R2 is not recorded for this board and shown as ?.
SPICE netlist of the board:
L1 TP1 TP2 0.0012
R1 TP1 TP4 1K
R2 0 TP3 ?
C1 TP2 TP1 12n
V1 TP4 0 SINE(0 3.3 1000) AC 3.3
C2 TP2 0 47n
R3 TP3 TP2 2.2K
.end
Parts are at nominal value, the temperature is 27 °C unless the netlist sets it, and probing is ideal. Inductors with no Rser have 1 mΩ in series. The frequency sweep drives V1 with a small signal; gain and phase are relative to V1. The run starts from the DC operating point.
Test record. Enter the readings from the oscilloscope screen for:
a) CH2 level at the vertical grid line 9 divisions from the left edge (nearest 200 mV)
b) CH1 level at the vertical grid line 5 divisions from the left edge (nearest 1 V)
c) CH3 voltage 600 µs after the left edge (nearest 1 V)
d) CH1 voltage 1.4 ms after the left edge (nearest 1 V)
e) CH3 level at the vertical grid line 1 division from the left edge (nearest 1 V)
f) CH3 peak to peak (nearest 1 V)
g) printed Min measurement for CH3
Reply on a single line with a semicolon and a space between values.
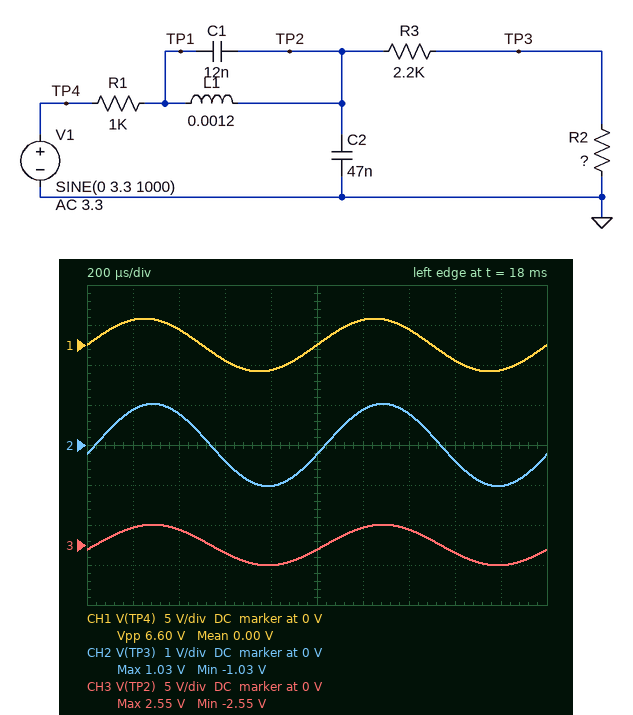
-1.0 V; 0 V; -1 V; 2 V; 2 V; 5 V; -2.55 V
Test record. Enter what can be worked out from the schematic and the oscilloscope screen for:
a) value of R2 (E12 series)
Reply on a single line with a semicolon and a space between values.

1.5 kΩ
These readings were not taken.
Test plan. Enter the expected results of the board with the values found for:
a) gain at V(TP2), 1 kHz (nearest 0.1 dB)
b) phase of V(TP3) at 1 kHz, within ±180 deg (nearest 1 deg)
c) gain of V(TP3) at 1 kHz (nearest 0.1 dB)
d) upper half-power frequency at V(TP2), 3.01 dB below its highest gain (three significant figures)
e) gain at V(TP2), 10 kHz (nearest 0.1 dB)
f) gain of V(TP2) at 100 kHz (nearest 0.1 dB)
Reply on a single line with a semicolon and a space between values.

-2.3 dB; -13 deg; -10.1 dB; 4.41 kHz; -10.0 dB; -29.6 dB
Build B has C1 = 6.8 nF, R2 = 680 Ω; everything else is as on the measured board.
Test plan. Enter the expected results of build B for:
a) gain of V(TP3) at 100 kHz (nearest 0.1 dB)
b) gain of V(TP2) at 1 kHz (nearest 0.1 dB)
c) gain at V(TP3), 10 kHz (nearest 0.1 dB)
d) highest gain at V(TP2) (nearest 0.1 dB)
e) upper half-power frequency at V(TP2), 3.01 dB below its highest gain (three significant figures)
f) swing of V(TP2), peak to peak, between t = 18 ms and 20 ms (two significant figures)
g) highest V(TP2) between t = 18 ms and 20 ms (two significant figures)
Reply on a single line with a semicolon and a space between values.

-42.5 dB; -2.8 dB; -22.6 dB; -2.6 dB; 4.68 kHz; 4.8 V; 2.4 V
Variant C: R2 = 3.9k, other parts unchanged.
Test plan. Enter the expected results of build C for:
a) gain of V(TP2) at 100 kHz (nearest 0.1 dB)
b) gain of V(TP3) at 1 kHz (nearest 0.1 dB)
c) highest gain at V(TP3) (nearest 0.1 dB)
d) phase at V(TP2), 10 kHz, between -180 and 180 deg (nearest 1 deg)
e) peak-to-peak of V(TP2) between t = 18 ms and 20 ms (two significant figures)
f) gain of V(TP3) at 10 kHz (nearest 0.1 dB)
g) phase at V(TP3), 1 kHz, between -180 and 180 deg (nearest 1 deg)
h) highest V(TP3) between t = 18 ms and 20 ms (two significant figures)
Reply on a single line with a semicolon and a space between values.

-29.6 dB; -5.5 dB; -5.2 dB; -73 deg; 5.5 V; -13.7 dB; -14 deg; 1.8 V
